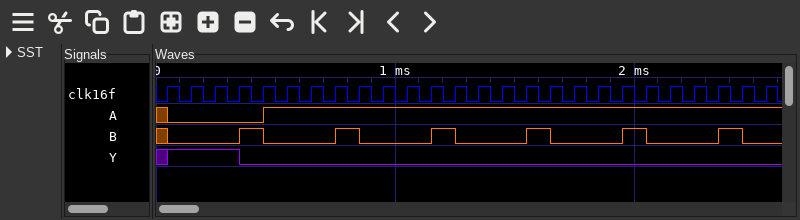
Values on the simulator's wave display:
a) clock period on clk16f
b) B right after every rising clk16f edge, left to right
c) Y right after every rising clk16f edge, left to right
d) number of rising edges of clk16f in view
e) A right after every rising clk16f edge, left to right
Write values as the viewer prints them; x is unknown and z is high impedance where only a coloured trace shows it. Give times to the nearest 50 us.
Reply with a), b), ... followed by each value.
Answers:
a) 100 us
b) 0 0 0 1 0 0 0 1 0 0 0 1 0 0 0 1 0 0 0 1 0 0 0 1 0 0
c) 1 1 1 0 0 0 0 0 0 0 0 0 0 0 0 0 0 0 0 0 0 0 0 0 0 0
d) 26
e) 0 0 0 0 1 1 1 1 1 1 1 1 1 1 1 1 1 1 1 1 1 1 1 1 1 1
